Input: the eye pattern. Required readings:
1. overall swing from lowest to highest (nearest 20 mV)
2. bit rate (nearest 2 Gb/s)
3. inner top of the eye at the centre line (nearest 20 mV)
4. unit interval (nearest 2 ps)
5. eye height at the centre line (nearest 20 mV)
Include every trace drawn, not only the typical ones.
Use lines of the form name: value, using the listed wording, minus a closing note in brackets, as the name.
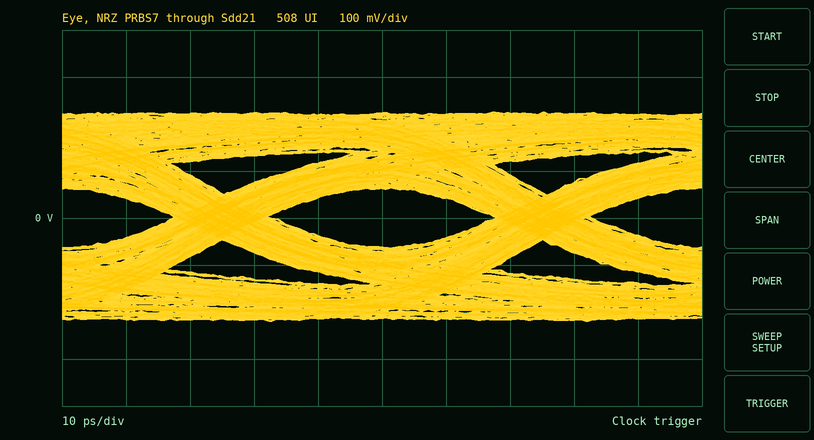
overall swing from lowest to highest: 440 mV
bit rate: 20 Gb/s
inner top of the eye at the centre line: 60 mV
unit interval: 50 ps
eye height at the centre line: 120 mV
